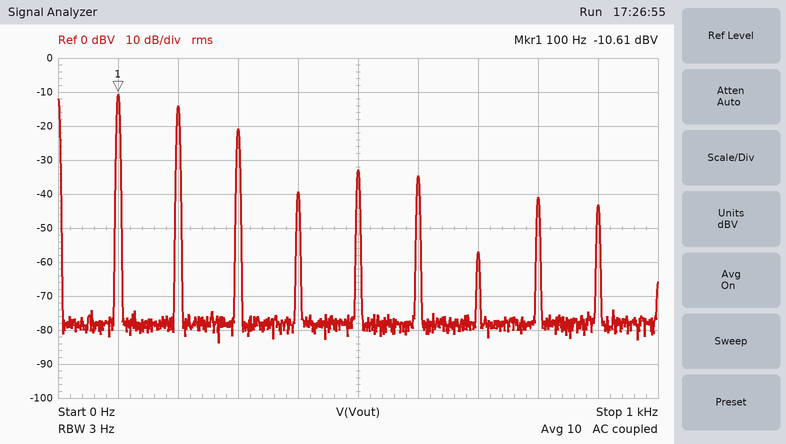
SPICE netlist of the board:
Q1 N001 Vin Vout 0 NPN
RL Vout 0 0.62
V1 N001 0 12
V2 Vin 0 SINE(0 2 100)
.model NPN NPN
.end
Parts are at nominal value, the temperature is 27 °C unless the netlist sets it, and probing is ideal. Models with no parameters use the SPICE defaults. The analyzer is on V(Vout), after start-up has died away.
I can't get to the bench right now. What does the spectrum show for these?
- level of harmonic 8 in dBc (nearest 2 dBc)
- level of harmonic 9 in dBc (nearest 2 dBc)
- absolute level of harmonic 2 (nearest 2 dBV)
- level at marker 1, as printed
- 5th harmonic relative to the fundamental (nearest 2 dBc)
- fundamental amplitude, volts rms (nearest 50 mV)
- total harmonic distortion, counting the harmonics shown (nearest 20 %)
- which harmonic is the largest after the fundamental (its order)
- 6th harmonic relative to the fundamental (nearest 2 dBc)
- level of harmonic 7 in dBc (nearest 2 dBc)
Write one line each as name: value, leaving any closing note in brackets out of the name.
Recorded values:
level of harmonic 8 in dBc: -30 dBc
level of harmonic 9 in dBc: -32 dBc
absolute level of harmonic 2: -14 dBV
level at marker 1, as printed: -10.61 dBV
5th harmonic relative to the fundamental: -22 dBc
fundamental amplitude, volts rms: 300 mV
total harmonic distortion, counting the harmonics shown: 80 %
which harmonic is the largest after the fundamental: 2
6th harmonic relative to the fundamental: -24 dBc
level of harmonic 7 in dBc: -46 dBc
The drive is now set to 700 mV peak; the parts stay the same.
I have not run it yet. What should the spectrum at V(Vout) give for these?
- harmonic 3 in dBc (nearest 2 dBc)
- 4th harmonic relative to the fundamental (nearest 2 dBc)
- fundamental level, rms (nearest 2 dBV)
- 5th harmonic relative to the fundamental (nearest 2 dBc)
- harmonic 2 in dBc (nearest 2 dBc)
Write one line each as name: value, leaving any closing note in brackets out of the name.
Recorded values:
harmonic 3 in dBc: -2 dBc
4th harmonic relative to the fundamental: -2 dBc
fundamental level, rms: -108 dBV
5th harmonic relative to the fundamental: -4 dBc
harmonic 2 in dBc: 0 dBc
